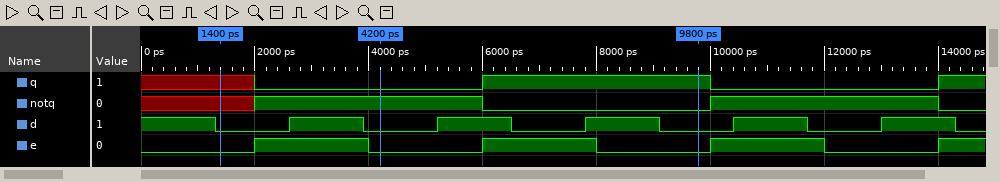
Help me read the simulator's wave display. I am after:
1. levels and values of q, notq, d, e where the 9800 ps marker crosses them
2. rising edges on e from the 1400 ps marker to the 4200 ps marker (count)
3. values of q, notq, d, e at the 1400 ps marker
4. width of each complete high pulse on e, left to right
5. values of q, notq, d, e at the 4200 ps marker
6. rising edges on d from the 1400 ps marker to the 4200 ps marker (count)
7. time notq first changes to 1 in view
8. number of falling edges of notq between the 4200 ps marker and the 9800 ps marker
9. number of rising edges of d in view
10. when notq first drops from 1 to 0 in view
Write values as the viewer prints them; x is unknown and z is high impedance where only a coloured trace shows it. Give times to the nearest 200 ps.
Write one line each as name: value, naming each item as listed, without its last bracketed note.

levels and values of q, notq, d, e where the 9800 ps marker crosses them: q=1, notq=0, d=0, e=0
rising edges on e from the 1400 ps marker to the 4200 ps marker: 1
values of q, notq, d, e at the 1400 ps marker: q=x, notq=x, d=0, e=0
width of each complete high pulse on e, left to right: 2000 ps, 2000 ps, 2000 ps
values of q, notq, d, e at the 4200 ps marker: q=0, notq=1, d=0, e=0
rising edges on d from the 1400 ps marker to the 4200 ps marker: 1
time notq first changes to 1 in view: 2000 ps
number of falling edges of notq between the 4200 ps marker and the 9800 ps marker: 1
number of rising edges of d in view: 5
when notq first drops from 1 to 0 in view: 6000 ps
